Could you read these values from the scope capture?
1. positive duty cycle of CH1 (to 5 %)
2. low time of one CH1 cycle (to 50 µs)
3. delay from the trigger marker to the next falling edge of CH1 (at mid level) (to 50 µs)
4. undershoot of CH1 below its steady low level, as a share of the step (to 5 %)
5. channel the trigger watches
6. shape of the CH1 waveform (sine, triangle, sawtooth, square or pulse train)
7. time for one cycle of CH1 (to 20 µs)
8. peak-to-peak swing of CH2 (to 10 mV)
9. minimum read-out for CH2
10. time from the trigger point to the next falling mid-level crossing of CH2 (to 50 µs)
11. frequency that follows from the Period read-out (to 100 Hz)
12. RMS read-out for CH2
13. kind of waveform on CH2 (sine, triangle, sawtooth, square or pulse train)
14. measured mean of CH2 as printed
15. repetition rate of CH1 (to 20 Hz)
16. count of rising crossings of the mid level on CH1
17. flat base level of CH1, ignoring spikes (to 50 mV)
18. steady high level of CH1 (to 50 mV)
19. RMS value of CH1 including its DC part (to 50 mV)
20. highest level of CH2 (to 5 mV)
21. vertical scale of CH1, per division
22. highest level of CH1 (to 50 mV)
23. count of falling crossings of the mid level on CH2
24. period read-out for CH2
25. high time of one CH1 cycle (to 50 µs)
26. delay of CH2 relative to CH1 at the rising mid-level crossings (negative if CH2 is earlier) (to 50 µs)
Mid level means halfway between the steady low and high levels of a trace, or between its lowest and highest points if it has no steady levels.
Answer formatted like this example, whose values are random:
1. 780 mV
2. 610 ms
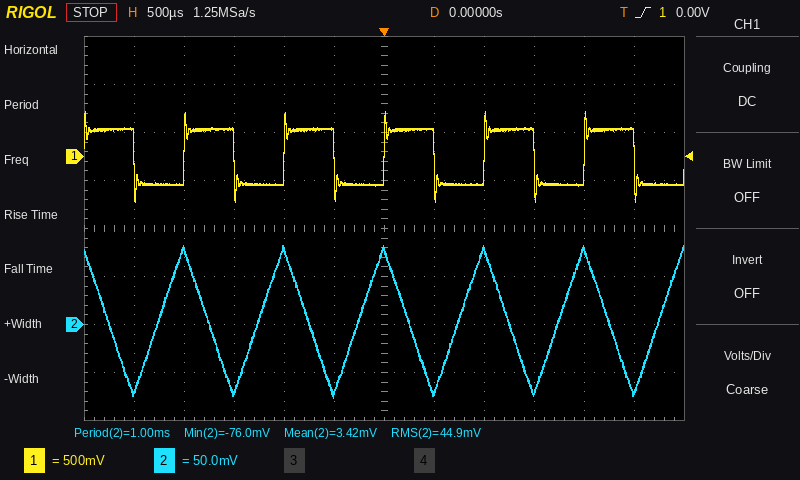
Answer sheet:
1. 50 %
2. 500 µs
3. 500 µs
4. 30 %
5. CH1
6. square
7. 1.00 ms
8. 160 mV
9. -76.0 mV
10. 250 µs
11. 1.0 kHz
12. 44.9 mV
13. triangle
14. 3.42 mV
15. 1.00 kHz
16. 5
17. -300 mV
18. 300 mV
19. 300 mV
20. 80 mV
21. 500 mV
22. 450 mV
23. 6
24. 1.00 ms
25. 500 µs
26. -250 µs
